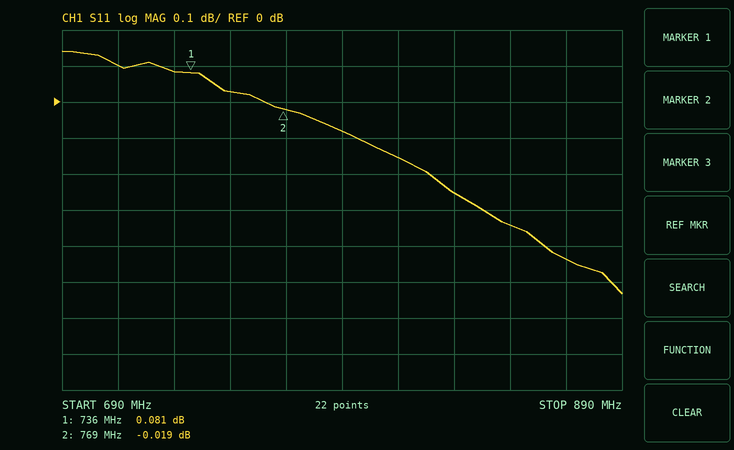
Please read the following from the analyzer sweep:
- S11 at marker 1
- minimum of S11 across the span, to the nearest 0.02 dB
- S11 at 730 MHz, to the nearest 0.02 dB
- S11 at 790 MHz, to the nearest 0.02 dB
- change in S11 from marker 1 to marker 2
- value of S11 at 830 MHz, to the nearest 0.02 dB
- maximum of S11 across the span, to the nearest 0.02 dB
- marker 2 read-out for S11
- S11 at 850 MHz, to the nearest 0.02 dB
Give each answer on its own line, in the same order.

0.081 dB
-0.54 dB
0.08 dB
-0.08 dB
-0.100 dB
-0.26 dB
0.14 dB
-0.019 dB
-0.34 dB
